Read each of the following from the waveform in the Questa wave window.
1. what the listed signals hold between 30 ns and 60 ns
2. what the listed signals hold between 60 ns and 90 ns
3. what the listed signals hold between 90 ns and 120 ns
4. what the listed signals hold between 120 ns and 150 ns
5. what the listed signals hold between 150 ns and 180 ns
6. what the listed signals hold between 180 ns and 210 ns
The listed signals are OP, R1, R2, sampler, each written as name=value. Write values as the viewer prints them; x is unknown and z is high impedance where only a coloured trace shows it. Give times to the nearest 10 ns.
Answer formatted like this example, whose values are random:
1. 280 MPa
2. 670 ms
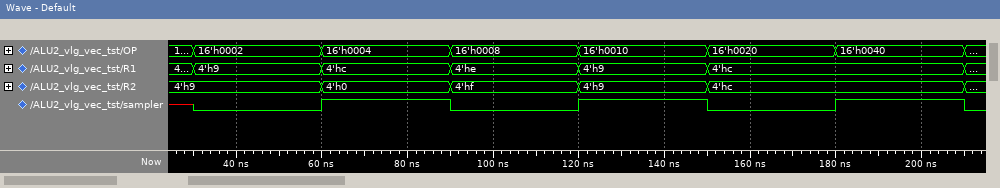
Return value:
1. OP=16'h0002, R1=4'h9, R2=4'h9, sampler=0
2. OP=16'h0004, R1=4'hc, R2=4'h0, sampler=1
3. OP=16'h0008, R1=4'he, R2=4'hf, sampler=0
4. OP=16'h0010, R1=4'h9, R2=4'h9, sampler=1
5. OP=16'h0020, R1=4'hc, R2=4'hc, sampler=0
6. OP=16'h0040, R1=4'hc, R2=4'hc, sampler=1
